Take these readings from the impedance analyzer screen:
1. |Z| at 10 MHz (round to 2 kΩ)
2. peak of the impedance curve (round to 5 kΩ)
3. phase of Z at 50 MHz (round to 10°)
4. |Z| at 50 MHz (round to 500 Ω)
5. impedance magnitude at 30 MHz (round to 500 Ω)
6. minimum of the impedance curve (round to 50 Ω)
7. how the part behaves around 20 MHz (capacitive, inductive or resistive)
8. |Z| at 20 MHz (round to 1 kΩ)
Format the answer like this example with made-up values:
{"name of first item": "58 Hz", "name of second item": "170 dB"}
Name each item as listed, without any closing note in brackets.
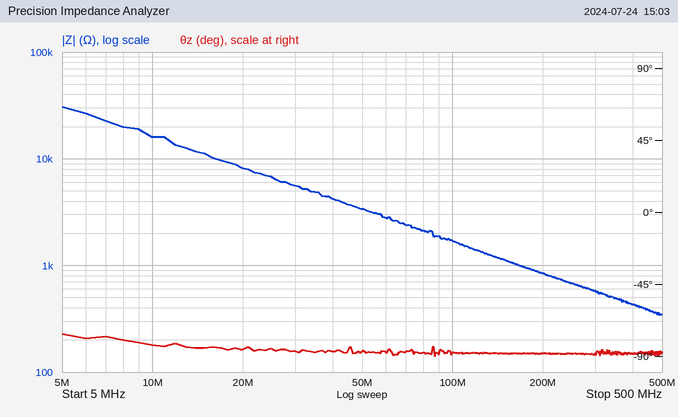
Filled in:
{"|Z| at 10 MHz": "16 kΩ", "peak of the impedance curve": "30 kΩ", "phase of Z at 50 MHz": "-90°", "|Z| at 50 MHz": "3.5 kΩ", "impedance magnitude at 30 MHz": "5.5 kΩ", "minimum of the impedance curve": "350 Ω", "how the part behaves around 20 MHz": "capacitive", "|Z| at 20 MHz": "8 kΩ"}
